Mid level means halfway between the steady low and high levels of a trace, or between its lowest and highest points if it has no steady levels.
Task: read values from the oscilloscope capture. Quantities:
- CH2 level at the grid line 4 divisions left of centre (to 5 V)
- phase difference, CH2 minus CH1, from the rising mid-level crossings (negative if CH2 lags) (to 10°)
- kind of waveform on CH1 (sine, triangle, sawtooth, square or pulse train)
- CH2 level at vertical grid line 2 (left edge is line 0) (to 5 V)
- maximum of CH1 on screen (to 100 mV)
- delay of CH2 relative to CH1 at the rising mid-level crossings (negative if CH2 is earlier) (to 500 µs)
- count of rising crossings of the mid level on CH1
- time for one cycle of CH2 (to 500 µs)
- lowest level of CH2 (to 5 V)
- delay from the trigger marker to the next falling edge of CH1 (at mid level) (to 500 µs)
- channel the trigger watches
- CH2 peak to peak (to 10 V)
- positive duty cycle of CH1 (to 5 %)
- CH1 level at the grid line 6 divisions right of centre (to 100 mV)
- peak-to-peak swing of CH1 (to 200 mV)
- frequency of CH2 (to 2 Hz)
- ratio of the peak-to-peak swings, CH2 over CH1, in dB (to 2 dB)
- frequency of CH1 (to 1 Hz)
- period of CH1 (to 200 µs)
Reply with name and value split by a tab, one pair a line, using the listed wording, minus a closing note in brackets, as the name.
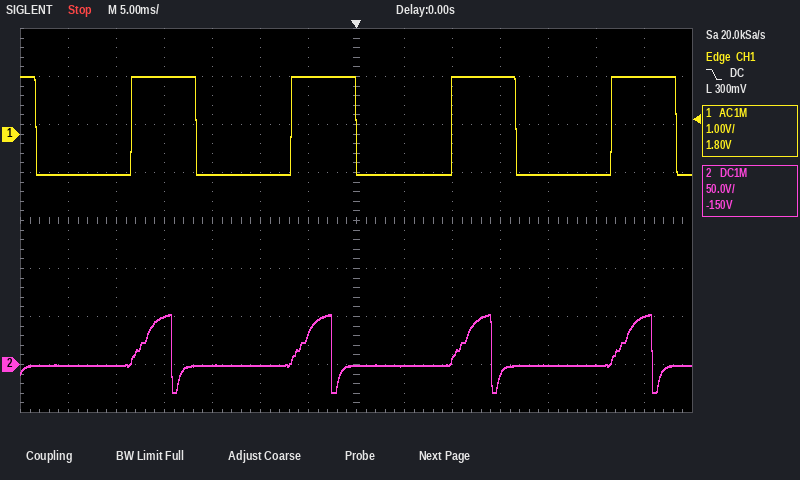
CH2 level at the grid line 4 divisions left of centre	50 V
phase difference, CH2 minus CH1, from the rising mid-level crossings (negative if CH2 lags)	-10°
kind of waveform on CH1	pulse train
CH2 level at vertical grid line 2 (left edge is line 0)	0 V
maximum of CH1 on screen	1.2 V
delay of CH2 relative to CH1 at the rising mid-level crossings (negative if CH2 is earlier)	+500 µs
count of rising crossings of the mid level on CH1	4
time for one cycle of CH2	16.5 ms
lowest level of CH2	-30 V
delay from the trigger marker to the next falling edge of CH1 (at mid level)	16.5 ms
channel the trigger watches	CH1
CH2 peak to peak	80 V
positive duty cycle of CH1	40 %
CH1 level at the grid line 6 divisions right of centre	1.2 V
peak-to-peak swing of CH1	2.0 V
frequency of CH2	60 Hz
ratio of the peak-to-peak swings, CH2 over CH1, in dB	32 dB
frequency of CH1	60 Hz
period of CH1	16.6 ms
